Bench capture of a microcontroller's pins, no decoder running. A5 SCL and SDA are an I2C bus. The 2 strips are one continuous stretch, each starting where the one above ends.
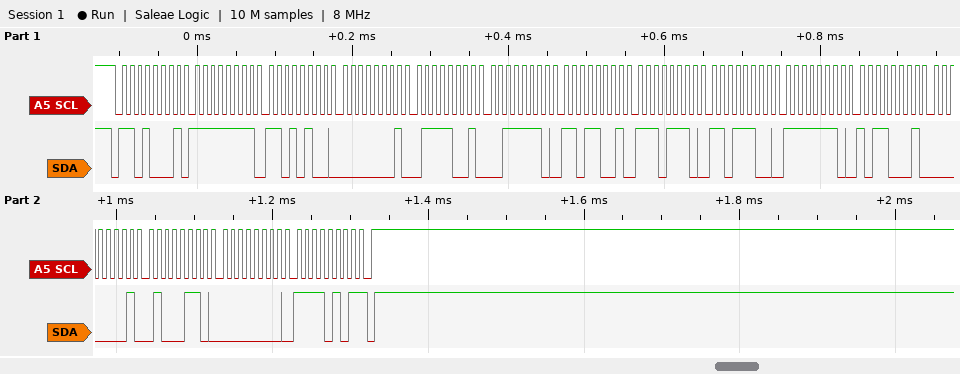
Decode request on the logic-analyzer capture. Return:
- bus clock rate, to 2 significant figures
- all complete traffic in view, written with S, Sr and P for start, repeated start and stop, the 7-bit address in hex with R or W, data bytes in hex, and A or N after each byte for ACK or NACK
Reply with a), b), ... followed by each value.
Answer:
a) 100 kHz
b) S 68R A FF A D4 A 01 A 79 A 3E A D9 A EE A DC A FE A B1 A 01 A 46 A 00 A F5 N P
